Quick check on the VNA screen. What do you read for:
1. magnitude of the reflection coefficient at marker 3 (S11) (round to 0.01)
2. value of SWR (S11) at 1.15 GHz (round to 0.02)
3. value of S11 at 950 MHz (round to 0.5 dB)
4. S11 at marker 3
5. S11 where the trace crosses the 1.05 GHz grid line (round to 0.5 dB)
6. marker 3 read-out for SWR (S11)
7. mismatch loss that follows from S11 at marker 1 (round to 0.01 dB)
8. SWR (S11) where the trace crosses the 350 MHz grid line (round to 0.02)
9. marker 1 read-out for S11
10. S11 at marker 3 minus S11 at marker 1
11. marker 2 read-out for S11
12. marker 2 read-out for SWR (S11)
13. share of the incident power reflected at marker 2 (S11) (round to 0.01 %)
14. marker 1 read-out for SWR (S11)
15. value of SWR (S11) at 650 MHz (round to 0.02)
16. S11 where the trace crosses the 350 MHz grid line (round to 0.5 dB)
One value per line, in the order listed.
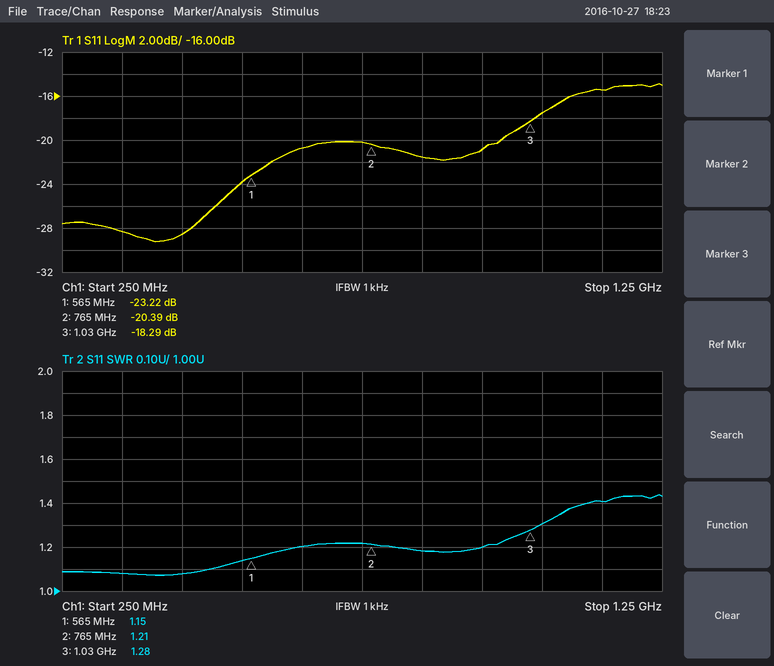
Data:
0.12
1.40
-21.0 dB
-18.29 dB
-17.5 dB
1.28
0.02 dB
1.08
-23.22 dB
4.93 dB
-20.39 dB
1.21
0.91 %
1.15
1.20
-28.5 dB
